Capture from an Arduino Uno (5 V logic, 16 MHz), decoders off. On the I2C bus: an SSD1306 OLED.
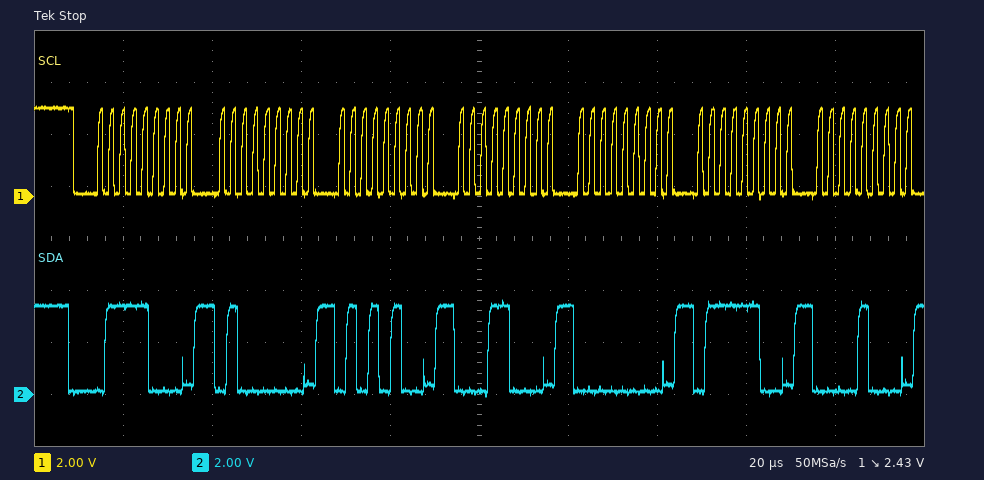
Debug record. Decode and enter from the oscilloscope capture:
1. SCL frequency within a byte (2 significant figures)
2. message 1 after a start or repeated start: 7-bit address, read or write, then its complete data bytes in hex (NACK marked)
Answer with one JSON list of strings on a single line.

["400 kHz", "0x3C write: 40 54 18 00 7C 08"]
